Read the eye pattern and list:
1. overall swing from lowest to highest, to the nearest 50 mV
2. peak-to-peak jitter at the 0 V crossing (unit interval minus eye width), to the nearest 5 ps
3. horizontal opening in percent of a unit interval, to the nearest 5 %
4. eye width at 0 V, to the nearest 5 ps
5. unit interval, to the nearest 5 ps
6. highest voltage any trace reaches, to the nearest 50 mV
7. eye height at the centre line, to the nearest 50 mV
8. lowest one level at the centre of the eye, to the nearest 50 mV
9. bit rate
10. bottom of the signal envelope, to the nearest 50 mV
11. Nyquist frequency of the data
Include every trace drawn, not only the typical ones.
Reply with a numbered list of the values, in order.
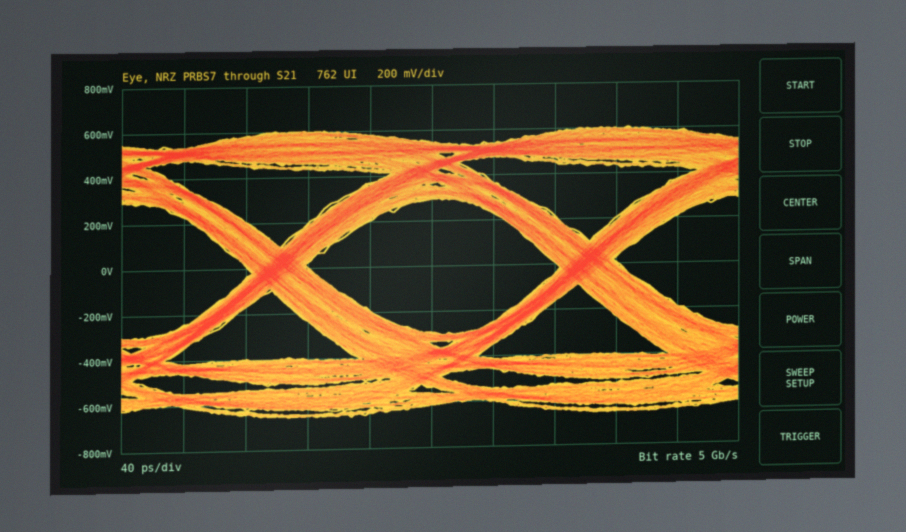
1. 1.25 V
2. 40 ps
3. 80 %
4. 160 ps
5. 200 ps
6. 600 mV
7. 600 mV
8. 300 mV
9. 5 Gb/s
10. -650 mV
11. 2.5 GHz
